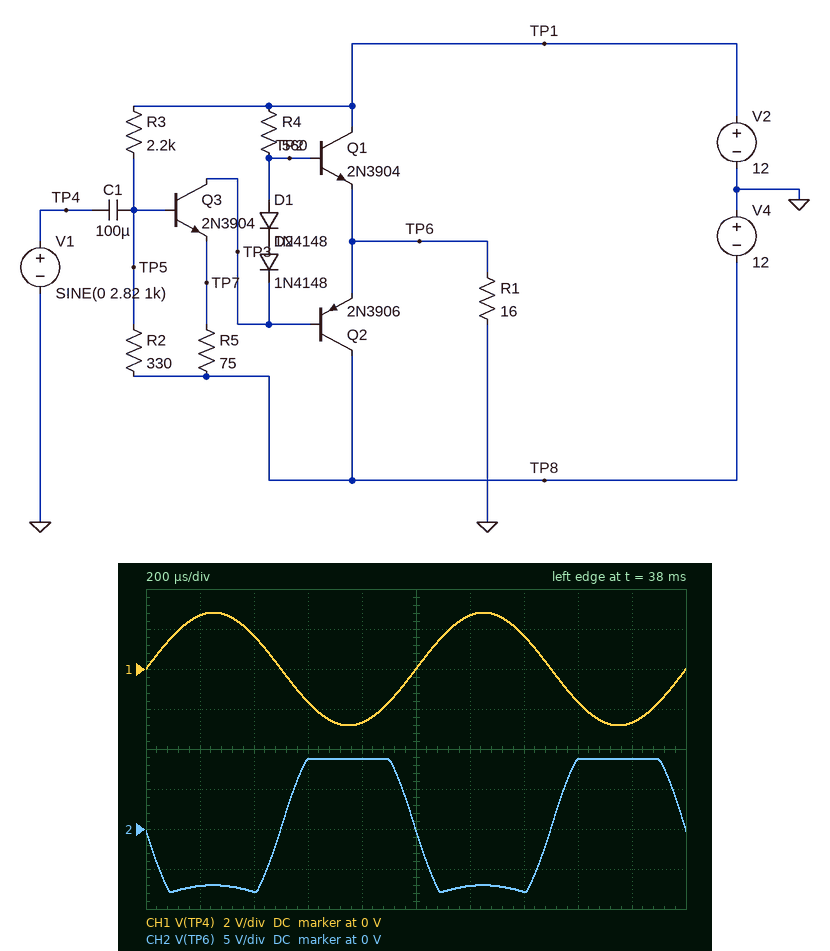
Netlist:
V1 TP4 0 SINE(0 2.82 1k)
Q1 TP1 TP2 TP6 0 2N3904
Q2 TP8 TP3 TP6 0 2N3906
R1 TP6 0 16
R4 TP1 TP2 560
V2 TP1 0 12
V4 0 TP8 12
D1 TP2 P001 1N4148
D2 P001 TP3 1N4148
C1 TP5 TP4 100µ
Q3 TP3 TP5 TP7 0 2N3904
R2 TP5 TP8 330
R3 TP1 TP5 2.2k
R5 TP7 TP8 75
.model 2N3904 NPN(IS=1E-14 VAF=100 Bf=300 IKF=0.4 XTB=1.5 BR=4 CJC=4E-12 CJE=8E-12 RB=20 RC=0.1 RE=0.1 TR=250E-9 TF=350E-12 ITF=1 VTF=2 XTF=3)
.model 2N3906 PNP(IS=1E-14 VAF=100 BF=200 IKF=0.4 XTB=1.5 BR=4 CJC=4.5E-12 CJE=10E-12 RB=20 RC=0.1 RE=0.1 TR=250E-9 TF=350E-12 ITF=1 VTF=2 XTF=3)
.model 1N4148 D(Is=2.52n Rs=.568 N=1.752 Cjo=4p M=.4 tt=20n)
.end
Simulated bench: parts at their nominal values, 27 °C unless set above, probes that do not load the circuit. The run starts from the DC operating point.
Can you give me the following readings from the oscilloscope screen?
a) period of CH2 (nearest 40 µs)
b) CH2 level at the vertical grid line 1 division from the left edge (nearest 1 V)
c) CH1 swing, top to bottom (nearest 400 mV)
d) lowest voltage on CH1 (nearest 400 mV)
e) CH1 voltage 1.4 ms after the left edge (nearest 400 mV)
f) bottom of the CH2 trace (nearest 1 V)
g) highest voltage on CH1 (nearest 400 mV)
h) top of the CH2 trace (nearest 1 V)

1.00 ms
-7 V
5.6 V
-2.8 V
1.6 V
-8 V
2.8 V
9 V
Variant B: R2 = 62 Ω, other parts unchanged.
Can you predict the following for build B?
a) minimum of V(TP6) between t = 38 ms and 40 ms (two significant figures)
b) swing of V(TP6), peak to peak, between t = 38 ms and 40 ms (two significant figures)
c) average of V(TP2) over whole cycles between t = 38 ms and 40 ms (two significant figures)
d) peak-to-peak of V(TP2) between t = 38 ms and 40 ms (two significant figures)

-6.6 V
15 V
4.7 V
16 V
